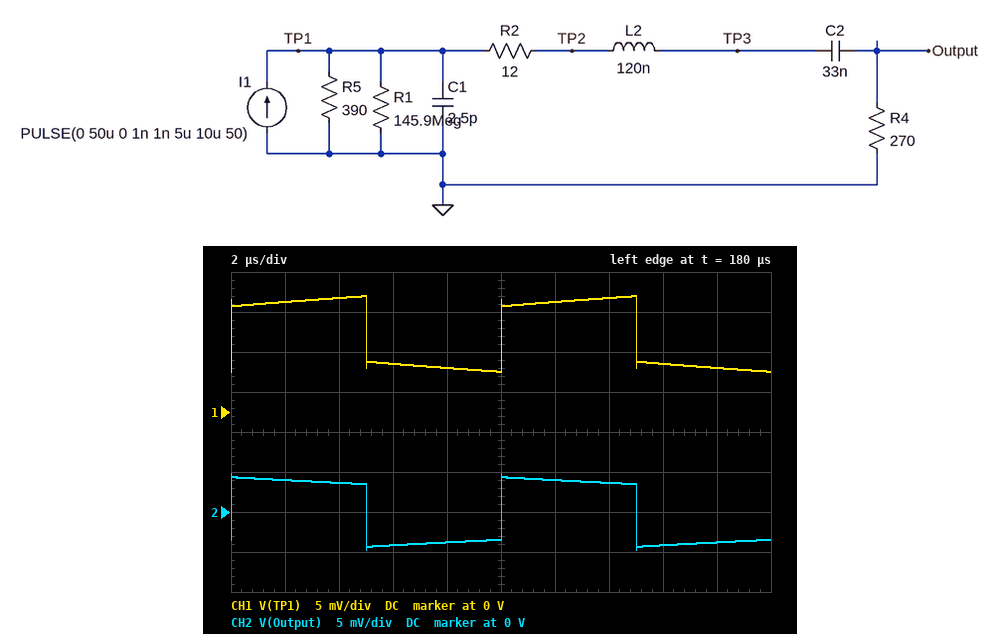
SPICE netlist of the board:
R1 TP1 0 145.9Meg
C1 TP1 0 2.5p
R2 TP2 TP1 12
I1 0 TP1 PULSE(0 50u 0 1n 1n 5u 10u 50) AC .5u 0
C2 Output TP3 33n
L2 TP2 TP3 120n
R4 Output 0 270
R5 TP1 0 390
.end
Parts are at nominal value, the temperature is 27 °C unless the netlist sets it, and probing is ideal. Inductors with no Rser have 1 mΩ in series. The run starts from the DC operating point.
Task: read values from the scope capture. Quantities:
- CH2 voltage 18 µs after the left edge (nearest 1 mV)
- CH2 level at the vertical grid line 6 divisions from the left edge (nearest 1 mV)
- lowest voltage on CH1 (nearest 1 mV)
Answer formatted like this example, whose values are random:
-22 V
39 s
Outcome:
-4 mV
4 mV
5 mV
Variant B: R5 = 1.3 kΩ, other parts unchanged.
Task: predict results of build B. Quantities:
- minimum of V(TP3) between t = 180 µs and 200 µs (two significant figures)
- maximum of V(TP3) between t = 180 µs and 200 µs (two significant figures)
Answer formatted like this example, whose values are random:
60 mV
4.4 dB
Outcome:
25 mV
39 mV
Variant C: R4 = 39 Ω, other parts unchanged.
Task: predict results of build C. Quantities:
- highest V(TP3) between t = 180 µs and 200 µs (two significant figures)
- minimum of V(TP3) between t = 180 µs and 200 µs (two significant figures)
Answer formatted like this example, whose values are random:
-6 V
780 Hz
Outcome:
12 mV
7.4 mV
